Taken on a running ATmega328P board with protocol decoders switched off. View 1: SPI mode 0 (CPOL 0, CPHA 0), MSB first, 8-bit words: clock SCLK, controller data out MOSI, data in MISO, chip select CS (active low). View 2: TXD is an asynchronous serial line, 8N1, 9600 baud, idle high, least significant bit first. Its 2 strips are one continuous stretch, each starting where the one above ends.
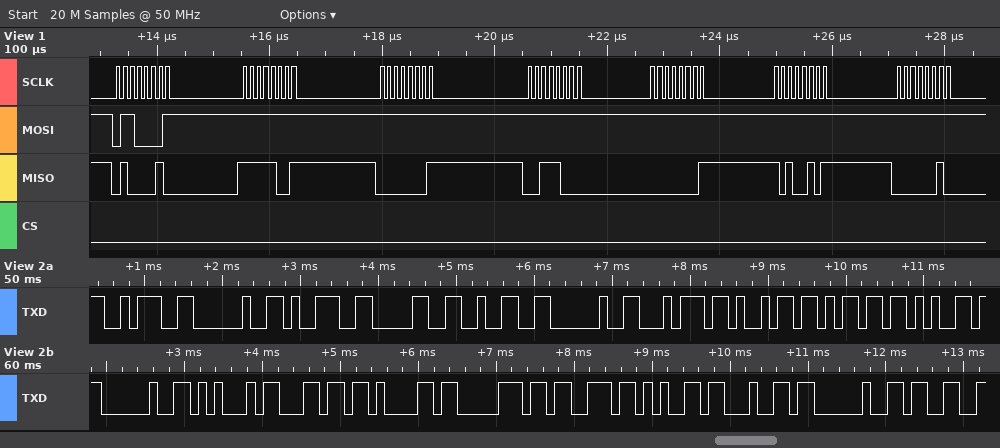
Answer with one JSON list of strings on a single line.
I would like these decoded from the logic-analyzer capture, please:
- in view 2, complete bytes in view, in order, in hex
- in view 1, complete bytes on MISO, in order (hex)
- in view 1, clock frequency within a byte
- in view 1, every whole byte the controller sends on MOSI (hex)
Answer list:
["0x3A 0x20 0x39 0x30 0x32 0x20 0x74 0x69 0x6D 0x65 0x20 0x45 0x6C 0x61 0x70 0x73 0x65 0x64 0x20 0x33", "42 F9 01 38 01 A5 02", "8 MHz", "61 FF FF FF FF FF FF"]
